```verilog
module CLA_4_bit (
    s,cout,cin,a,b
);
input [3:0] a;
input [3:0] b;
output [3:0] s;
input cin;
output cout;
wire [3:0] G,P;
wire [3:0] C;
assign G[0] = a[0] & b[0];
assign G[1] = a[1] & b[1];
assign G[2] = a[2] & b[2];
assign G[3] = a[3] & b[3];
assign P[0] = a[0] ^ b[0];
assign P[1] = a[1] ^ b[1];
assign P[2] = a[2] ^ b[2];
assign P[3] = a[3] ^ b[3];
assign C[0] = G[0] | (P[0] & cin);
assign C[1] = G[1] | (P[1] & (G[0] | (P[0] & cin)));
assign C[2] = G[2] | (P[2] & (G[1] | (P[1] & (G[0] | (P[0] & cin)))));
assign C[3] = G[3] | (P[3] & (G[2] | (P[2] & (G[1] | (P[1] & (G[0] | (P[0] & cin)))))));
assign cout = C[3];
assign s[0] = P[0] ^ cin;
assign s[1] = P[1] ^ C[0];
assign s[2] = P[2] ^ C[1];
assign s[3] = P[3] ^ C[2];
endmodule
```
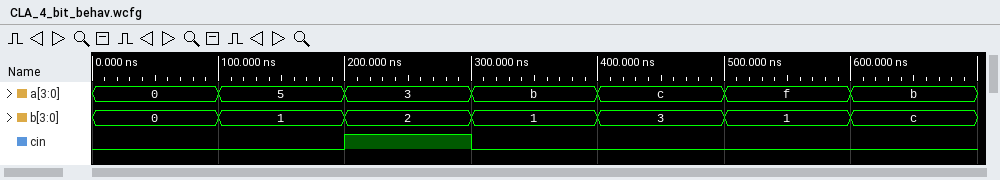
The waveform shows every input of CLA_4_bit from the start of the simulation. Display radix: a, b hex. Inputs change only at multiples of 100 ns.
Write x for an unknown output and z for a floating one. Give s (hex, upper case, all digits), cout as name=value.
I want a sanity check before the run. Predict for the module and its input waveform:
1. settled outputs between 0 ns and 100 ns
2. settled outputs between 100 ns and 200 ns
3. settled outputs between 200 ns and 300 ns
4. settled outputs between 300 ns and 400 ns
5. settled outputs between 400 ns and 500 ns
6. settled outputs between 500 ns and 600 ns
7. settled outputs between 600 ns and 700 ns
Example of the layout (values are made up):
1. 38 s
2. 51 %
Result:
1. s=0, cout=0
2. s=6, cout=0
3. s=6, cout=0
4. s=C, cout=0
5. s=F, cout=0
6. s=0, cout=1
7. s=7, cout=1
